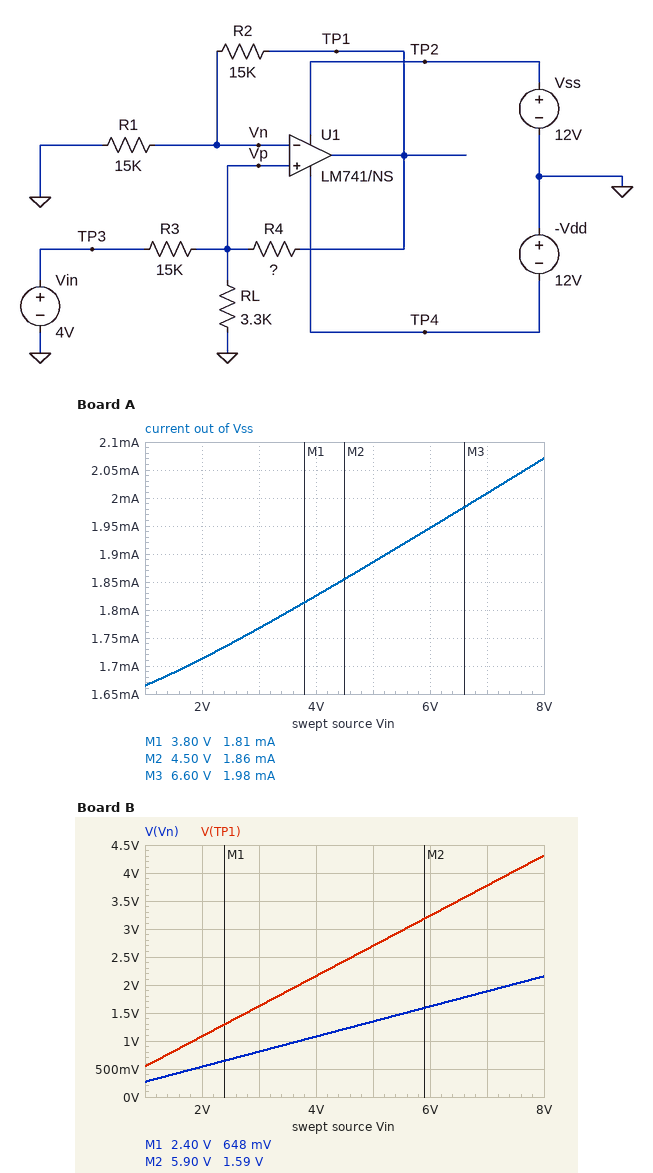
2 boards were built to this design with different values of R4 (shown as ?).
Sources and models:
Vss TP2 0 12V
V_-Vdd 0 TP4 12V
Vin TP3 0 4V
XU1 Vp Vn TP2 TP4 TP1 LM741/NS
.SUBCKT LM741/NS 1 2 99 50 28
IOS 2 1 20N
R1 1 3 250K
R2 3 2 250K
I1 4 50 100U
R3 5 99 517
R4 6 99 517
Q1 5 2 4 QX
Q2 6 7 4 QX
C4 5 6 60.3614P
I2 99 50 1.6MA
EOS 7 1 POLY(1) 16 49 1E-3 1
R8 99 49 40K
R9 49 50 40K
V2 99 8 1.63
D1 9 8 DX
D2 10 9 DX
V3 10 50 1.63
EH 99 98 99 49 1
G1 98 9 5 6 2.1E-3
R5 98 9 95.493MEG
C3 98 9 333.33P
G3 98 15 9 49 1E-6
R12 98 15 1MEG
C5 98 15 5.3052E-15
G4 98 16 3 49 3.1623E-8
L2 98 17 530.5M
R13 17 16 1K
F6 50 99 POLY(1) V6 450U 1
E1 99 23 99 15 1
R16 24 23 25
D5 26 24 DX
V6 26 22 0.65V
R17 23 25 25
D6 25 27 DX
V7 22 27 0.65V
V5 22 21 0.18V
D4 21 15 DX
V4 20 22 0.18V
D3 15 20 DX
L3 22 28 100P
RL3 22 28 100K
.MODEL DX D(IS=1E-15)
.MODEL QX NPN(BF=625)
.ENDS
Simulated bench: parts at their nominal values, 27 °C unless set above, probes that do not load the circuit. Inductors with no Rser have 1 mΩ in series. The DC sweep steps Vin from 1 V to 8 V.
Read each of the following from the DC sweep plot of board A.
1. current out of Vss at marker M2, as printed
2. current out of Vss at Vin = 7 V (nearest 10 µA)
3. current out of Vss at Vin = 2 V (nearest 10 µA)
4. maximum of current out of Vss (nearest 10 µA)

1.86 mA
2.01 mA
1.71 mA
2.07 mA
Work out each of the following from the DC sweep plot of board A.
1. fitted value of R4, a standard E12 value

6.8 kΩ
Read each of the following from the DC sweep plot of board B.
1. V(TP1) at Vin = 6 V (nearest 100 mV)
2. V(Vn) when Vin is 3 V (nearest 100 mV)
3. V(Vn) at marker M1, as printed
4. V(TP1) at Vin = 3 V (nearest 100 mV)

3.2 V
800 mV
648 mV
1.6 V
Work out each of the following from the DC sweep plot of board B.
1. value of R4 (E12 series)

8.2 kΩ
